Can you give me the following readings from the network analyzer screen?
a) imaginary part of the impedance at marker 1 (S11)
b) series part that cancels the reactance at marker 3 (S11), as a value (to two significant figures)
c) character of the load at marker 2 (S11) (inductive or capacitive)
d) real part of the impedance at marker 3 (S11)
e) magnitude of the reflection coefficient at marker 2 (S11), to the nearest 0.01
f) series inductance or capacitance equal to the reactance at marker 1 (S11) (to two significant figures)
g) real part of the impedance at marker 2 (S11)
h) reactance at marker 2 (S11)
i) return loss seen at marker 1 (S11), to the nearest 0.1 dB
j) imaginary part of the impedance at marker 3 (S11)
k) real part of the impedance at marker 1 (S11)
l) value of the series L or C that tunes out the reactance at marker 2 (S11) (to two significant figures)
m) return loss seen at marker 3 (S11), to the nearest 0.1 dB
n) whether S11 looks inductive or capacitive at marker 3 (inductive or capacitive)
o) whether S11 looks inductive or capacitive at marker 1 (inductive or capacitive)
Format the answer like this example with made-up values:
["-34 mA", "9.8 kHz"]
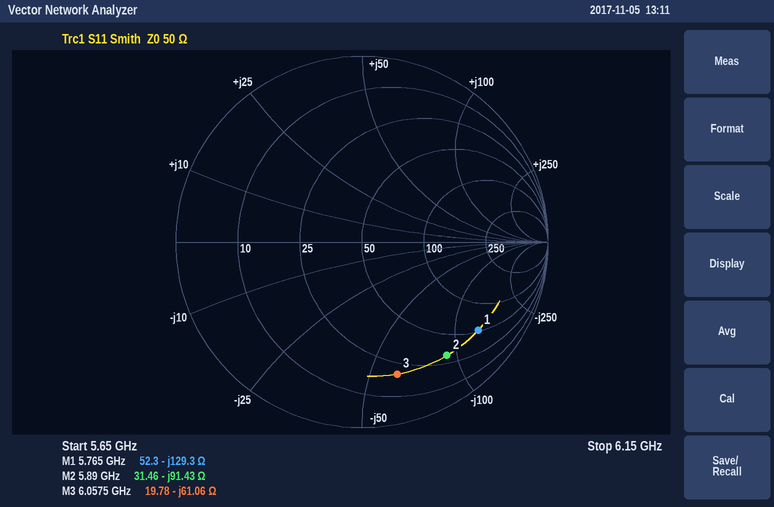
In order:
["-129.3 Ω", "1.6 nH", "capacitive", "19.78 Ω", "0.76", "210 fF", "31.46 Ω", "-91.43 Ω", "2.1 dB", "-61.06 Ω", "52.3 Ω", "2.5 nH", "2.7 dB", "capacitive", "capacitive"]
